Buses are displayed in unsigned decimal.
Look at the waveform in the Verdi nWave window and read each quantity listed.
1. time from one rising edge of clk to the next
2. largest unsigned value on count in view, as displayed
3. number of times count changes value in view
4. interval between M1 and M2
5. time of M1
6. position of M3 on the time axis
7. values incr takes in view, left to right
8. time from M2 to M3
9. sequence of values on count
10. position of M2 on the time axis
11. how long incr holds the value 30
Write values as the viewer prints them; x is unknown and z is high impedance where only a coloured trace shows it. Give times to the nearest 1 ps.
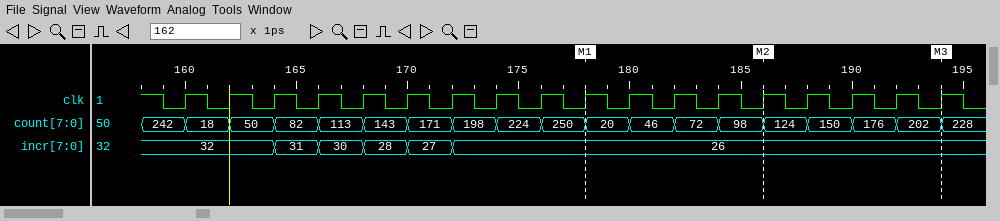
2 ps
250
18
8 ps
178 ps
194 ps
32, 31, 30, 28, 27, 26
8 ps
242, 18, 50, 82, 113, 143, 171, 198, 224, 250, 20, 46, 72, 98, 124, 150, 176, 202, 228
186 ps
2 ps
